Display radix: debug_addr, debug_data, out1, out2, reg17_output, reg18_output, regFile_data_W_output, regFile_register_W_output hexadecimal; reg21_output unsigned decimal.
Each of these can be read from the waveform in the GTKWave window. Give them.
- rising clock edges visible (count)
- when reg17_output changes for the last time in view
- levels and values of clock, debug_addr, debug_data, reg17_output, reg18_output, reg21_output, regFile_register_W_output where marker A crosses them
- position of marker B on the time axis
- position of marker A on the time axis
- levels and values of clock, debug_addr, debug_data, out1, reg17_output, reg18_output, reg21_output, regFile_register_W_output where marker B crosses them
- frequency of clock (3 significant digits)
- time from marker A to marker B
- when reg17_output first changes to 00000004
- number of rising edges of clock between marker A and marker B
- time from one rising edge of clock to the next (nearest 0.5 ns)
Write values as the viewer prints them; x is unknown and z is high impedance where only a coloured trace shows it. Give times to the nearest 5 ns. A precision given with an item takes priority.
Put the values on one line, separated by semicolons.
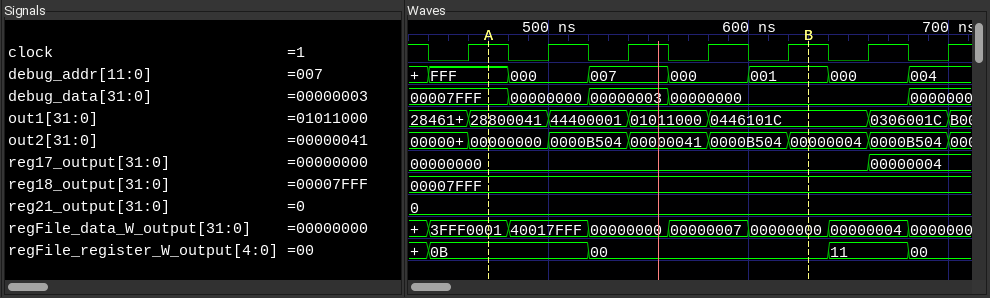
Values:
7; 660 ns; clock=1, debug_addr=FFF, debug_data=00007FFF, reg17_output=00000000, reg18_output=00007FFF, reg21_output=0, regFile_register_W_output=0B; 630 ns; 470 ns; clock=1, debug_addr=001, debug_data=00000000, out1=0446101C, reg17_output=00000000, reg18_output=00007FFF, reg21_output=0, regFile_register_W_output=00; 25.0 MHz; 160 ns; 660 ns; 4; 40 ns
